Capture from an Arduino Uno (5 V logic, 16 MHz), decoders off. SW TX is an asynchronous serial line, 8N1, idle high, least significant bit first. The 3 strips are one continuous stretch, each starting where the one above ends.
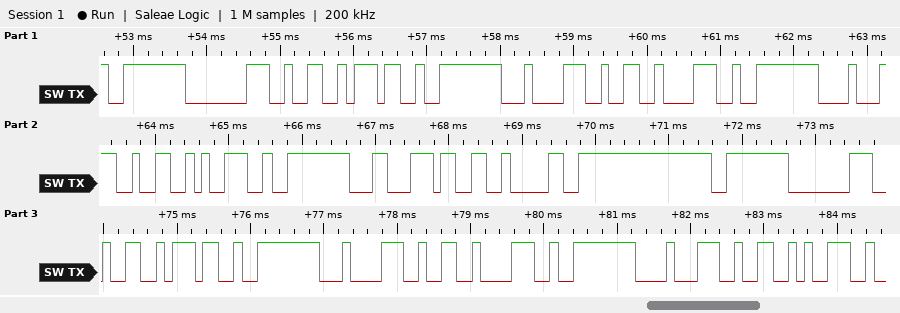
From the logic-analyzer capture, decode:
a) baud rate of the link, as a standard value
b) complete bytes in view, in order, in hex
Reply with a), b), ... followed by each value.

a) 9600 baud
b) FE 80 32 37 FE 84 32 38 FE 88 32 39 FE 8C 33 30 FE 80 32 37 FE 84 32 38 FE 88 32 39
